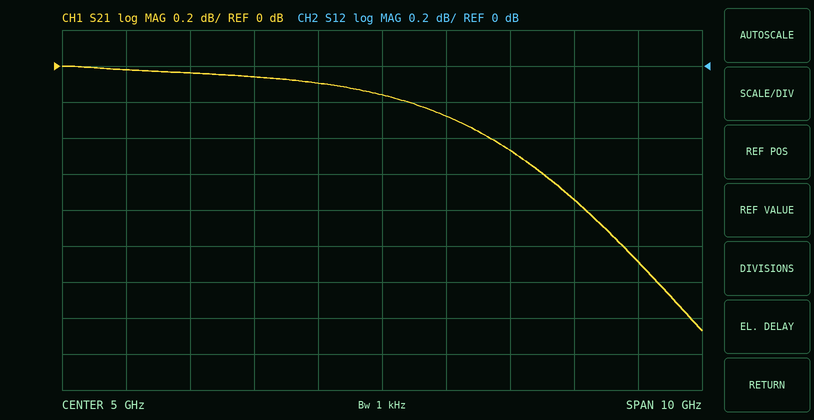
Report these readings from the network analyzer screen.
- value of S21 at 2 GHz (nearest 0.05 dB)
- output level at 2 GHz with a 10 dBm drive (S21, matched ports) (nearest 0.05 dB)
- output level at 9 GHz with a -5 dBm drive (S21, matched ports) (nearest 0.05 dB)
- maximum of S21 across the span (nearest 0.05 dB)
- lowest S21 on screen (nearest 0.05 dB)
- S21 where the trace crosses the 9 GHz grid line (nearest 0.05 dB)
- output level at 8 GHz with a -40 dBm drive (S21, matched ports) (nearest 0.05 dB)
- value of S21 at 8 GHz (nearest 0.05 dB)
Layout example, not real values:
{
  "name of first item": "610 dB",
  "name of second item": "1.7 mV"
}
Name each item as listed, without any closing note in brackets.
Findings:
{
  "value of S21 at 2 GHz": "-0.05 dB",
  "output level at 2 GHz with a 10 dBm drive (S21, matched ports)": "9.95 dBm",
  "output level at 9 GHz with a -5 dBm drive (S21, matched ports)": "-6.10 dBm",
  "maximum of S21 across the span": "0.00 dB",
  "lowest S21 on screen": "-1.45 dB",
  "S21 where the trace crosses the 9 GHz grid line": "-1.10 dB",
  "output level at 8 GHz with a -40 dBm drive (S21, matched ports)": "-40.75 dBm",
  "value of S21 at 8 GHz": "-0.75 dB"
}
